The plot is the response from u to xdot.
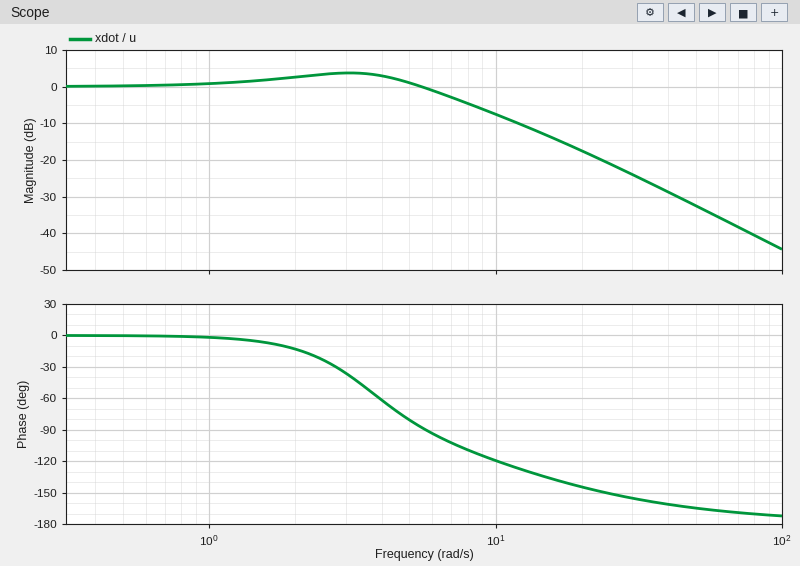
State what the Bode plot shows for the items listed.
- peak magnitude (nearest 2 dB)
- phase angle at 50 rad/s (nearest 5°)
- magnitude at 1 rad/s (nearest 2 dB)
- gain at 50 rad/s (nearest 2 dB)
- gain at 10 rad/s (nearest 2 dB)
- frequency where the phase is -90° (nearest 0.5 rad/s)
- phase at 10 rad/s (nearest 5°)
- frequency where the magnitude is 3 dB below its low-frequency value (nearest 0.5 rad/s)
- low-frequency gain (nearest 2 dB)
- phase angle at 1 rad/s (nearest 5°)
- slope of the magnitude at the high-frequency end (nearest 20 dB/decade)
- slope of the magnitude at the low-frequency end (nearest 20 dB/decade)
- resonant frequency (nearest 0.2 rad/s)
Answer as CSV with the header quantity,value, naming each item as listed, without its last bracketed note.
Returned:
quantity,value
peak magnitude,4 dB
phase angle at 50 rad/s,-165°
magnitude at 1 rad/s,0 dB
gain at 50 rad/s,-32 dB
gain at 10 rad/s,-8 dB
frequency where the phase is -90°,5.5 rad/s
phase at 10 rad/s,-120°
frequency where the magnitude is 3 dB below its low-frequency value,7.0 rad/s
low-frequency gain,0 dB
phase angle at 1 rad/s,0°
slope of the magnitude at the high-frequency end,-40 dB/decade
slope of the magnitude at the low-frequency end,0 dB/decade
resonant frequency,3.0 rad/s
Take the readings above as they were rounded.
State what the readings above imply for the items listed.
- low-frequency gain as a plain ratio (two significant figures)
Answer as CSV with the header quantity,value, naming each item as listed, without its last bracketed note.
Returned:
quantity,value
low-frequency gain as a plain ratio,1.0
